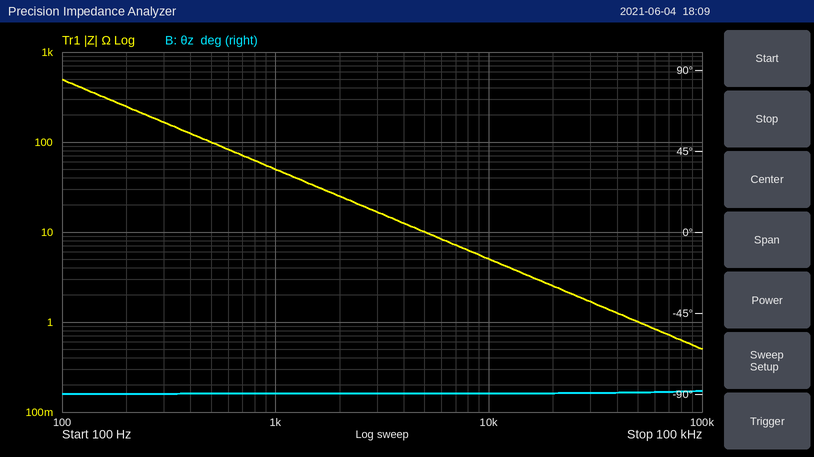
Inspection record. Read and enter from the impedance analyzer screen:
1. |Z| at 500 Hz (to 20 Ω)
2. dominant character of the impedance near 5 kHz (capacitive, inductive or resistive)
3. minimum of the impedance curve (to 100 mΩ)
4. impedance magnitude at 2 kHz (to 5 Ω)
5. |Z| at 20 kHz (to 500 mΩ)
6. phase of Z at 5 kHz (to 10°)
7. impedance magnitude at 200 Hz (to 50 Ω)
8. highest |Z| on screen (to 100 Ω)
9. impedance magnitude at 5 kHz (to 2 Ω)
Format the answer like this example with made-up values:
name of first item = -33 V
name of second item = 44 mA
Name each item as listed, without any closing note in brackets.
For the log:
|Z| at 500 Hz = 100 Ω
dominant character of the impedance near 5 kHz = capacitive
minimum of the impedance curve = 500 mΩ
impedance magnitude at 2 kHz = 25 Ω
|Z| at 20 kHz = 2.5 Ω
phase of Z at 5 kHz = -90°
impedance magnitude at 200 Hz = 250 Ω
highest |Z| on screen = 500 Ω
impedance magnitude at 5 kHz = 10 Ω
